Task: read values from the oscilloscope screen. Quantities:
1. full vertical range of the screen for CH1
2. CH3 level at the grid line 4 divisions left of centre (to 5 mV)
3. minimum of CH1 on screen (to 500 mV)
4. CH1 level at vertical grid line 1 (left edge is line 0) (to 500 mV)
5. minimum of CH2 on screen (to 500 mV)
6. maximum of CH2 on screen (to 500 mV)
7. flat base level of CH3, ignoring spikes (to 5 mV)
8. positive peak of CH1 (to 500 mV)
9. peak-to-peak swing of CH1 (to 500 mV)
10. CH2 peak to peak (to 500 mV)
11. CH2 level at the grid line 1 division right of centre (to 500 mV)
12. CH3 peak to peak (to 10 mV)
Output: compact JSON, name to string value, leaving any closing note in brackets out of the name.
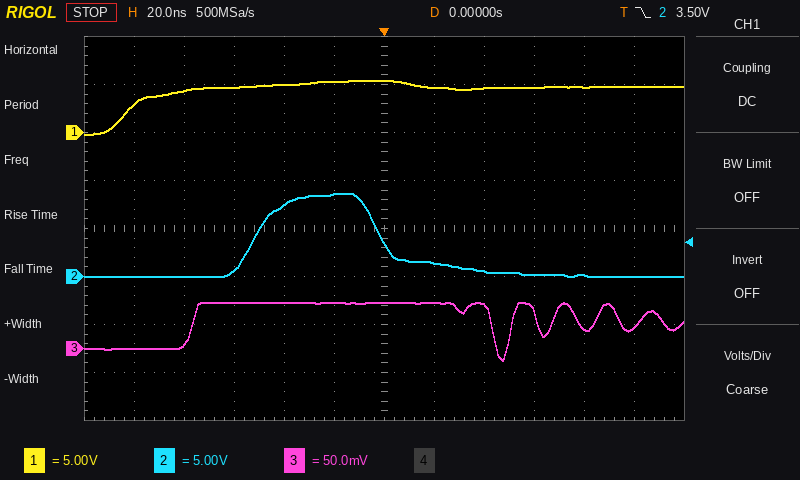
{"full vertical range of the screen for CH1": "40 V", "CH3 level at the grid line 4 divisions left of centre": "5 mV", "minimum of CH1 on screen": "0.0 V", "CH1 level at vertical grid line 1 (left edge is line 0)": "3.0 V", "minimum of CH2 on screen": "0.0 V", "maximum of CH2 on screen": "8.5 V", "flat base level of CH3, ignoring spikes": "0 mV", "positive peak of CH1": "5.5 V", "peak-to-peak swing of CH1": "5.5 V", "CH2 peak to peak": "8.5 V", "CH2 level at the grid line 1 division right of centre": "1.5 V", "CH3 peak to peak": "60 mV"}
